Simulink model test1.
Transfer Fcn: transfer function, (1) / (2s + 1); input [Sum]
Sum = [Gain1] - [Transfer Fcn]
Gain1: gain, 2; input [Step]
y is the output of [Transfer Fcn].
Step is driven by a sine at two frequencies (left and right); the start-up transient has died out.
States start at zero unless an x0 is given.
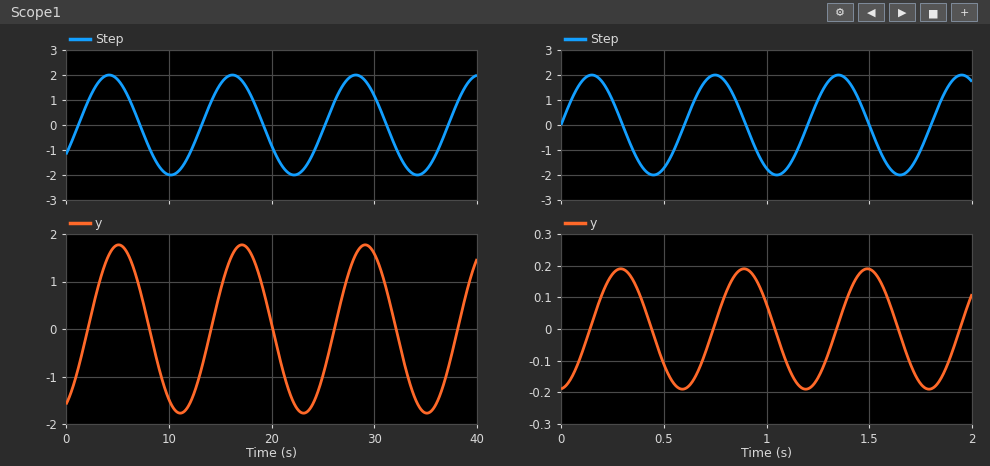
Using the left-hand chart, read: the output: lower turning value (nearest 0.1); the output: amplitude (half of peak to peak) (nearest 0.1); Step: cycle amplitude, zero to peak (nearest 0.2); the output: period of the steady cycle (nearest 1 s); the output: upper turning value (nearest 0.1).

-1.8
1.8
2.0
12 s
1.8
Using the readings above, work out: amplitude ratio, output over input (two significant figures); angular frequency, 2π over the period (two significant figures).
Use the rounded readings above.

0.90
0.52 rad/s
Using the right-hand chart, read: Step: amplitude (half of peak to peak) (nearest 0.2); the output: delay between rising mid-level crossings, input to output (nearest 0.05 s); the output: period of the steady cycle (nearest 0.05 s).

2.0
0.15 s
0.60 s
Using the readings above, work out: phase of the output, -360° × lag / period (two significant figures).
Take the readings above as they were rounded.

-90°
